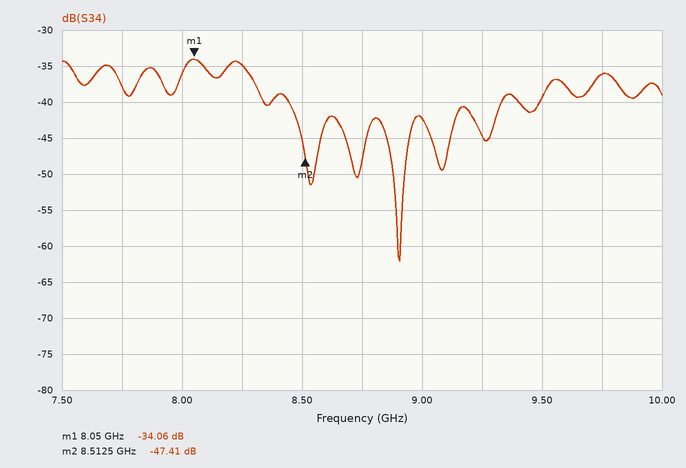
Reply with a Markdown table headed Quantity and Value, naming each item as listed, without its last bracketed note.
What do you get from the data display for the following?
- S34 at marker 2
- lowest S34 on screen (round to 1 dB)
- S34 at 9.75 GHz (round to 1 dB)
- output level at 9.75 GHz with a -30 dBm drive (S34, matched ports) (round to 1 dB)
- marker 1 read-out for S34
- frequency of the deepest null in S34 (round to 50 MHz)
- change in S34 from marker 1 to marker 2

| Quantity | Value |
|---|---|
| S34 at marker 2 | -47.41 dB |
| lowest S34 on screen | -62 dB |
| S34 at 9.75 GHz | -36 dB |
| output level at 9.75 GHz with a -30 dBm drive (S34, matched ports) | -66 dBm |
| marker 1 read-out for S34 | -34.06 dB |
| frequency of the deepest null in S34 | 8.90 GHz |
| change in S34 from marker 1 to marker 2 | -13.35 dB |
